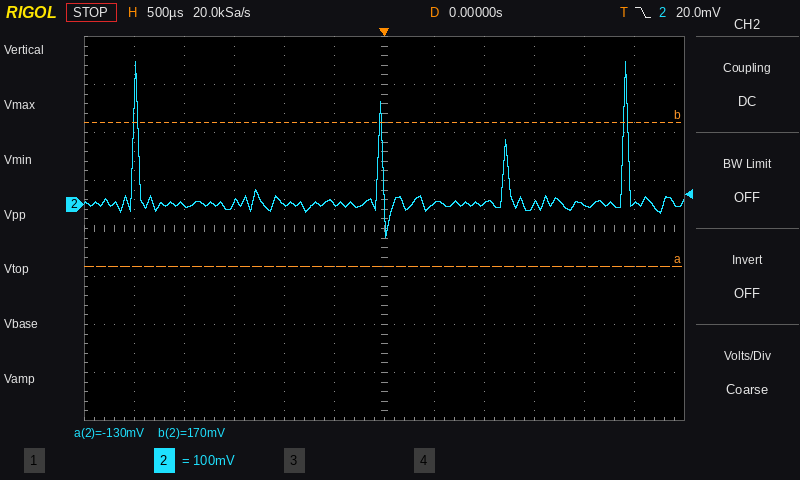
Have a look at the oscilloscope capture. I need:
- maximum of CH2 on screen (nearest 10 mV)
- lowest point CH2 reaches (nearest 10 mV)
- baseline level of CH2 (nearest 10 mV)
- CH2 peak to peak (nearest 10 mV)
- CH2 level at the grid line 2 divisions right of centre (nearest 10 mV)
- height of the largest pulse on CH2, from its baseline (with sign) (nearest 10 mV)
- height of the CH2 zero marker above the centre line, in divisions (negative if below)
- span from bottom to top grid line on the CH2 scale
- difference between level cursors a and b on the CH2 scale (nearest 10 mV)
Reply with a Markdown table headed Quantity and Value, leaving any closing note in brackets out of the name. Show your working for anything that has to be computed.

| Quantity | Value |
|---|---|
| maximum of CH2 on screen | 300 mV |
| lowest point CH2 reaches | -70 mV |
| baseline level of CH2 | 0 mV |
| CH2 peak to peak | 300 mV − (-70 mV) = 370 mV |
| CH2 level at the grid line 2 divisions right of centre | 0 mV |
| height of the largest pulse on CH2, from its baseline (with sign) | 300 mV − (0 mV) = +300 mV |
| height of the CH2 zero marker above the centre line, in divisions | +0.5 div |
| span from bottom to top grid line on the CH2 scale | 800 mV |
| difference between level cursors a and b on the CH2 scale | 300 mV |
